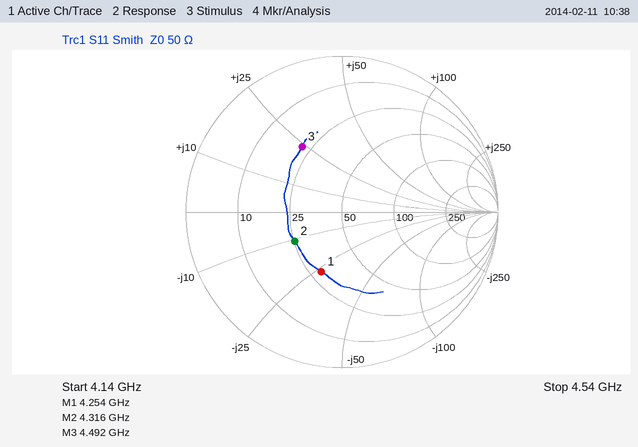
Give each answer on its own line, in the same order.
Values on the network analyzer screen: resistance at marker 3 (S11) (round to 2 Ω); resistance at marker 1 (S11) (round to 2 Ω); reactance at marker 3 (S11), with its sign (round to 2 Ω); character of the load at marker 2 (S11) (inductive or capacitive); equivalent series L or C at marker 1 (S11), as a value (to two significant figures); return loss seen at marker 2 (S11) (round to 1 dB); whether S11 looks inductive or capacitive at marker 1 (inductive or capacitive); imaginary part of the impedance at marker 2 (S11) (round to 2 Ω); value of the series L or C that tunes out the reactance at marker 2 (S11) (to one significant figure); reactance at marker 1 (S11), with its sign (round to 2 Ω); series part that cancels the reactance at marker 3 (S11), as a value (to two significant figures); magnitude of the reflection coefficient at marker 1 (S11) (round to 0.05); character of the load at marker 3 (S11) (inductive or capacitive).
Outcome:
22 Ω
30 Ω
+24 Ω
capacitive
1.4 pF
9 dB
capacitive
-10 Ω
400 pH
-26 Ω
1.5 pF
0.40
inductive
